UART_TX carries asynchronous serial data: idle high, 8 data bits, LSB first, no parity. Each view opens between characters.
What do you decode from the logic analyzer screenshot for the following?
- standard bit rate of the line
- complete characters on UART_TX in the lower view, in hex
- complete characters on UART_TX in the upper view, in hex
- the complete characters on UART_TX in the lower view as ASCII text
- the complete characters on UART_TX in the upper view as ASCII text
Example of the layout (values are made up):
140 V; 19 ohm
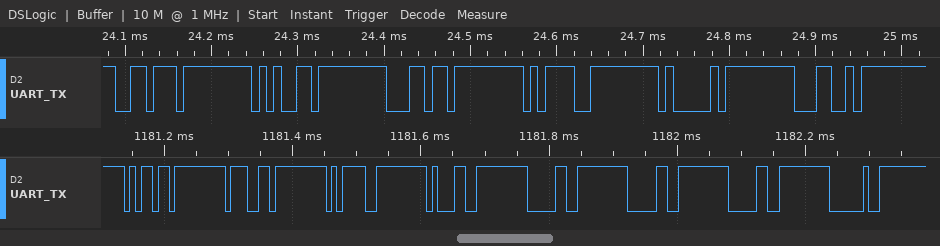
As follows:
115200 baud; 6D, 67, 3D, 31, 30, 30, 30, 20; 76, 65, 6C, 3D, 41, 4C; "mg=1000 "; "vel=AL"
